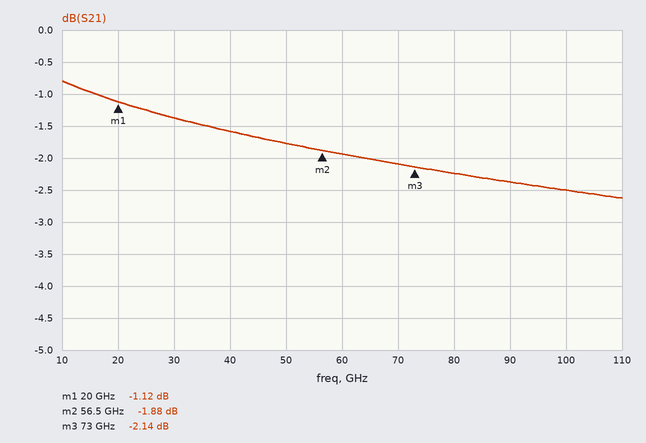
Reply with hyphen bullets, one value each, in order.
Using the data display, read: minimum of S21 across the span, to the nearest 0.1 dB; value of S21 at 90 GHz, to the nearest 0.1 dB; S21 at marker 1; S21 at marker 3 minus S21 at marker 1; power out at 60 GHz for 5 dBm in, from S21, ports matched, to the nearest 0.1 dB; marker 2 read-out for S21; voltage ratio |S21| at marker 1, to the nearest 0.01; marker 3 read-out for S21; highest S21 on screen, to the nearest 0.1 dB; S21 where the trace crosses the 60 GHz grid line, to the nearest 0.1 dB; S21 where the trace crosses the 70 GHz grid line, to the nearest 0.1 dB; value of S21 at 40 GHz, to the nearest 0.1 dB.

- -2.6 dB
- -2.4 dB
- -1.12 dB
- -1.02 dB
- 3.1 dBm
- -1.88 dB
- 0.88
- -2.14 dB
- -0.8 dB
- -1.9 dB
- -2.1 dB
- -1.6 dB
